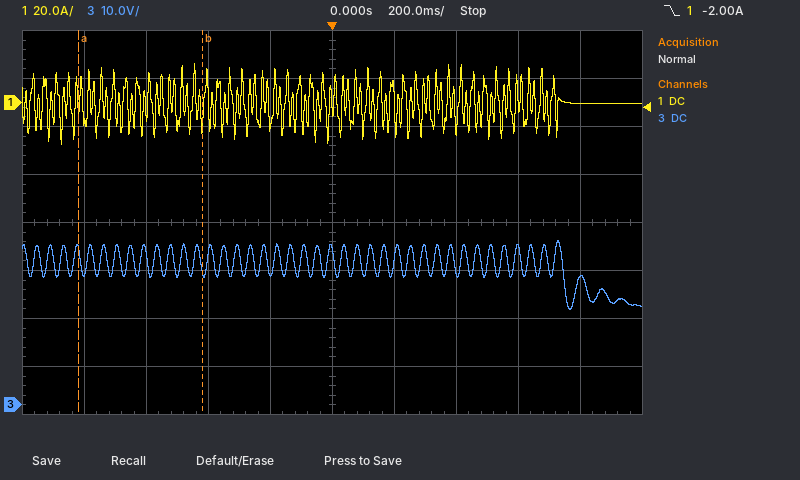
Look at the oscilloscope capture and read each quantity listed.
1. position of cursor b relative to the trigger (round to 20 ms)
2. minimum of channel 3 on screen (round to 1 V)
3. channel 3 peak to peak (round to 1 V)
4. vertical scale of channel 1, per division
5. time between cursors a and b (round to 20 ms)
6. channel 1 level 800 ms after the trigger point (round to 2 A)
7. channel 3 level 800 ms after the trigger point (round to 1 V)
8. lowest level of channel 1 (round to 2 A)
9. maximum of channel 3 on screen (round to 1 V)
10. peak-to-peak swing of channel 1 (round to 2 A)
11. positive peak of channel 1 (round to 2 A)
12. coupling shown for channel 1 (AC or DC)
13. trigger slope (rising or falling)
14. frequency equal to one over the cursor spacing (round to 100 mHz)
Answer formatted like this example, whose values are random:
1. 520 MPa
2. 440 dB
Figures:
1. -420 ms
2. 20 V
3. 14 V
4. 20 A
5. 400 ms
6. 0 A
7. 26 V
8. -18 A
9. 34 V
10. 34 A
11. 16 A
12. DC
13. falling
14. 2.5 Hz
